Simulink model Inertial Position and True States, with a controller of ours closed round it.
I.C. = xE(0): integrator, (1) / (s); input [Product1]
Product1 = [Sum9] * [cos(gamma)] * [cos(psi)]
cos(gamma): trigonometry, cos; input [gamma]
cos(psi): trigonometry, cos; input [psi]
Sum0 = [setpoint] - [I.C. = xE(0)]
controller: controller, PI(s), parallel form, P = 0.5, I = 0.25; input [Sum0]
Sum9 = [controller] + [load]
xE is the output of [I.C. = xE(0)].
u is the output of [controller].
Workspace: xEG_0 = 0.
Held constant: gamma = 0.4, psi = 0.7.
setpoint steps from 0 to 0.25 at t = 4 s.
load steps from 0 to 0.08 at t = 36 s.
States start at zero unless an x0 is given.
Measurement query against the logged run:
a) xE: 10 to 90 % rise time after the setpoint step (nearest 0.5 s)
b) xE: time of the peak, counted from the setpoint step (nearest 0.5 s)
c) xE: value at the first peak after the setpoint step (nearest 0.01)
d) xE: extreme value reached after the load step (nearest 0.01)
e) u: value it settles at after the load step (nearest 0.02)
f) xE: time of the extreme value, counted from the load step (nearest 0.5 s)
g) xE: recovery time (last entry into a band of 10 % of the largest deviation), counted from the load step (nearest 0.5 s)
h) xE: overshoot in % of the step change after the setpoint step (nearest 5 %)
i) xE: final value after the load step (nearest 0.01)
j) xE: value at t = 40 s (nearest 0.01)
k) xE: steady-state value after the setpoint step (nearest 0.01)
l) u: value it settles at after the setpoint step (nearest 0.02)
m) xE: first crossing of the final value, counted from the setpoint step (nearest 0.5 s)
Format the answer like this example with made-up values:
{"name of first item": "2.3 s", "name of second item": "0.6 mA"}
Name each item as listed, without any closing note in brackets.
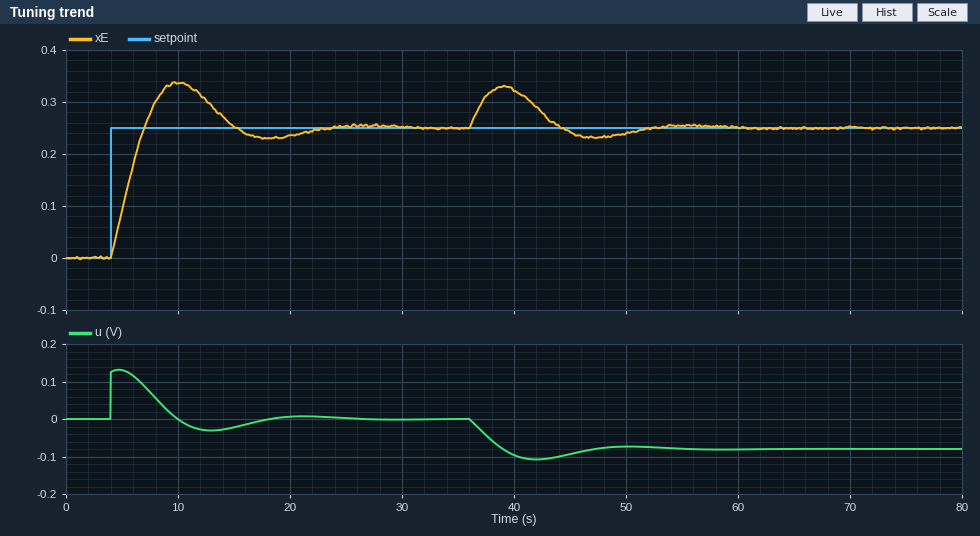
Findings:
{"xE: 10 to 90 % rise time after the setpoint step": "2.5 s", "xE: time of the peak, counted from the setpoint step": "6.0 s", "xE: value at the first peak after the setpoint step": "0.34", "xE: extreme value reached after the load step": "0.33", "u: value it settles at after the load step": "-0.08", "xE: time of the extreme value, counted from the load step": "3.0 s", "xE: recovery time (last entry into a band of 10 % of the largest deviation), counted from the load step": "14.5 s", "xE: overshoot in % of the step change after the setpoint step": "35 %", "xE: final value after the load step": "0.25", "xE: value at t = 40 s": "0.32", "xE: steady-state value after the setpoint step": "0.25", "u: value it settles at after the setpoint step": "0.00", "xE: first crossing of the final value, counted from the setpoint step": "3.0 s"}
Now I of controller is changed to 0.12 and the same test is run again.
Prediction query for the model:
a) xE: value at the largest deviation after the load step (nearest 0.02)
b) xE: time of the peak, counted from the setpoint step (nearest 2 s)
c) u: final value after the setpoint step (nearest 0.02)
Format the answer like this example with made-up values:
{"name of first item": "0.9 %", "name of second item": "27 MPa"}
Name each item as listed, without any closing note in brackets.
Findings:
{"xE: value at the largest deviation after the load step": "0.34", "xE: time of the peak, counted from the setpoint step": "8 s", "u: final value after the setpoint step": "0.00"}
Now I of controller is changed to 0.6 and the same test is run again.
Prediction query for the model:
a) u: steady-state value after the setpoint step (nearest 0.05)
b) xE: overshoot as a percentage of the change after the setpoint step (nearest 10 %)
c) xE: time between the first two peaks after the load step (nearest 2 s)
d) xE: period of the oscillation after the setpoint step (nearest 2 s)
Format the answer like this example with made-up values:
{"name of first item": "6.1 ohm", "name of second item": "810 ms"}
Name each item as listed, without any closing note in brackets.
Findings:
{"u: steady-state value after the setpoint step": "0.00", "xE: overshoot as a percentage of the change after the setpoint step": "50 %", "xE: time between the first two peaks after the load step": "10 s", "xE: period of the oscillation after the setpoint step": "10 s"}
